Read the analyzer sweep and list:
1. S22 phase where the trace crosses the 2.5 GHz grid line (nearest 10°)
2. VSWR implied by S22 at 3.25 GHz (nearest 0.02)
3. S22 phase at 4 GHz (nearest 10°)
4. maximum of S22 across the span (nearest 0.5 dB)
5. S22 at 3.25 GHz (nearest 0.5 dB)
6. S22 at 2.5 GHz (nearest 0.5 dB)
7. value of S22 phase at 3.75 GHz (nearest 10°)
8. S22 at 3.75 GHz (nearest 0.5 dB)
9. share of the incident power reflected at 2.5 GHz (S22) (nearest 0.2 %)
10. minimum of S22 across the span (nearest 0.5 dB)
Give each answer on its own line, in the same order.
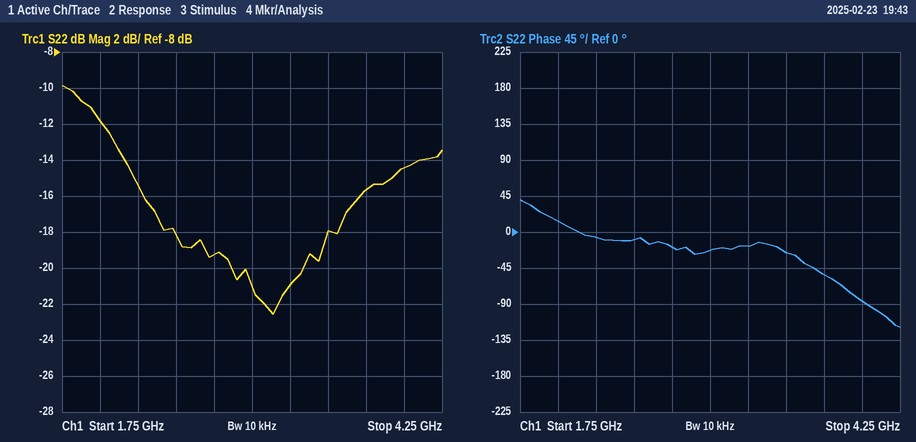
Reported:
-10°
1.20
-90°
-10.0 dB
-21.0 dB
-18.0 dB
-50°
-15.5 dB
1.6 %
-22.5 dB
